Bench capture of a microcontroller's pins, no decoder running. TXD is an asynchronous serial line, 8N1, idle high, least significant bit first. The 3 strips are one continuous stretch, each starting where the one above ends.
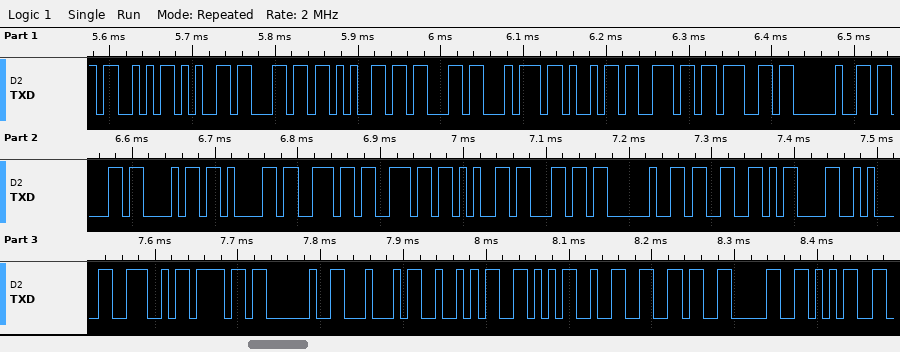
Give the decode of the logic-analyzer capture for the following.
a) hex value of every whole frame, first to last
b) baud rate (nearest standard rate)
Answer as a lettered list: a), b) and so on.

a) 53 65 6C 65 63 74 69 6E 67 20 63 68 61 6E 6E 65 6C 20 33 0D 0A 4E 6F 20 44 52 56 32 36 30 35
b) 115200 baud
